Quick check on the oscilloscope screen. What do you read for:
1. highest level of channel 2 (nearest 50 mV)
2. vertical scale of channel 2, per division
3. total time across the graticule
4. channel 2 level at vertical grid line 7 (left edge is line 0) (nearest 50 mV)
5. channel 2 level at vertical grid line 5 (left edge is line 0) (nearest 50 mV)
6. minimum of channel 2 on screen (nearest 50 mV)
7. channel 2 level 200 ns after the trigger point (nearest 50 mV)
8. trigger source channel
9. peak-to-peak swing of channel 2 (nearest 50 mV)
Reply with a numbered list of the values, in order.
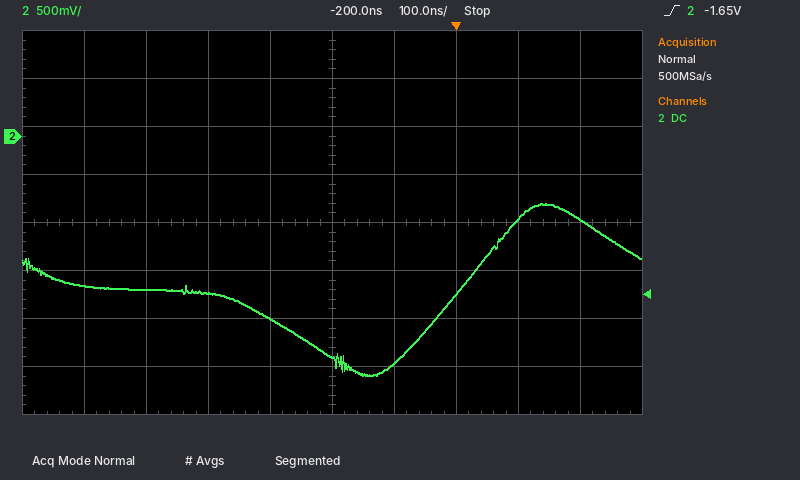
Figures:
1. -700 mV
2. 500 mV
3. 1 µs
4. -1.65 V
5. -2.30 V
6. -2.50 V
7. -850 mV
8. channel 2
9. 1.80 V
